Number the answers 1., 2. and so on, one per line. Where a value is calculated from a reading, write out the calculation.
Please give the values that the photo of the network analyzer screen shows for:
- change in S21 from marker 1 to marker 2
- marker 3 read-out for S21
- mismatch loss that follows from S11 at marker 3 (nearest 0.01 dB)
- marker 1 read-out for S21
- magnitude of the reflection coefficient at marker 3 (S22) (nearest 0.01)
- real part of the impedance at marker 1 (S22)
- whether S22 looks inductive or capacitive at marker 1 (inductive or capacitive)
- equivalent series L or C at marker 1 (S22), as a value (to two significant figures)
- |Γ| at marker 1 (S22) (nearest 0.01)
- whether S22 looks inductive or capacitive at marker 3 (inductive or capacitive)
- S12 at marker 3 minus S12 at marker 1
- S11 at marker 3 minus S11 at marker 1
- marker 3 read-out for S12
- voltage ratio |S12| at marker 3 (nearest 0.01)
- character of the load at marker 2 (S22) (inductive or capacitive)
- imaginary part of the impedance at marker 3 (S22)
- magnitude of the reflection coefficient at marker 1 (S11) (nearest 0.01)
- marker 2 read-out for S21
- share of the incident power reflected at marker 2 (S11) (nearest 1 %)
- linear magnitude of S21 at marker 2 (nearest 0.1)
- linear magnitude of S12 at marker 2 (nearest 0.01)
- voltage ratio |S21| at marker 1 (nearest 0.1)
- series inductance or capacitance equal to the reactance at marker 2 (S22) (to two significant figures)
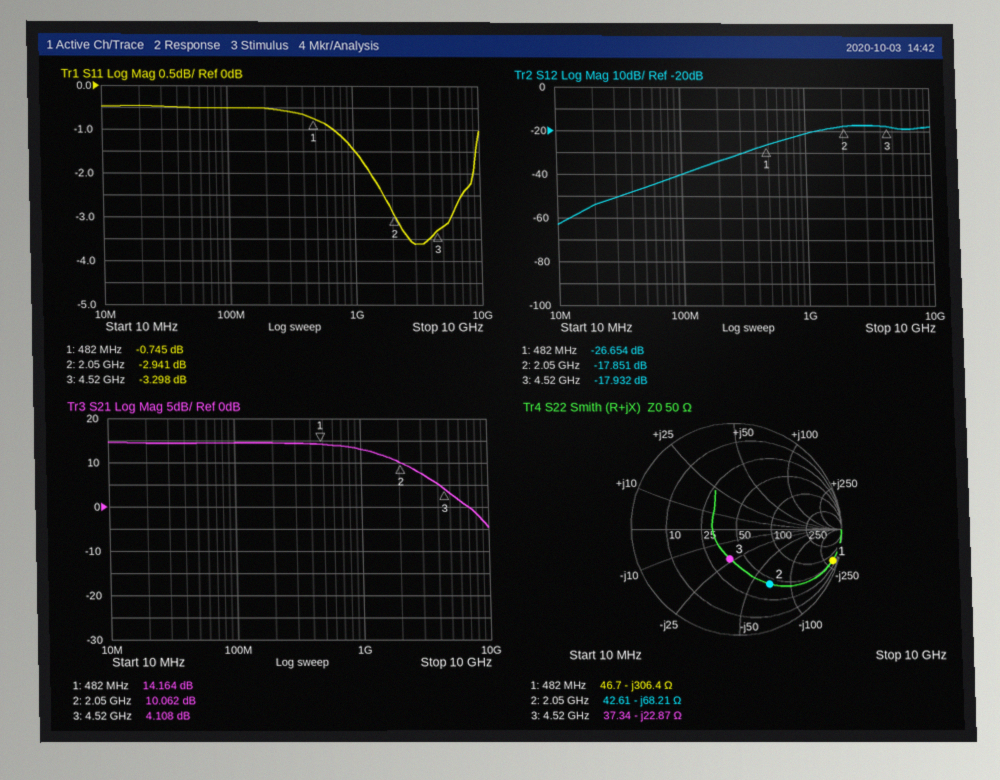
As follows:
1. 10.062 − (14.164) = -4.102 dB
2. 4.108 dB
3. −10 log10(1 − 10^(-3.298/10)) ≈ 2.74 dB
4. 14.164 dB
5. 0.29
6. 46.7 Ω
7. capacitive
8. C = 1/(2π × 482 MHz × 306.4 Ω) ≈ 1.1 pF
9. 0.95
10. capacitive
11. -17.932 − (-26.654) = 8.722 dB
12. -3.298 − (-0.745) = -2.553 dB
13. -17.932 dB
14. 10^(-17.932/20) ≈ 0.13
15. capacitive
16. -22.87 Ω
17. 10^(-0.745/20) ≈ 0.92
18. 10.062 dB
19. 10^(-2.941/10) ≈ 51 %
20. 10^(10.062/20) ≈ 3.2
21. 10^(-17.851/20) ≈ 0.13
22. 10^(14.164/20) ≈ 5.1
23. C = 1/(2π × 2.05 GHz × 68.21 Ω) ≈ 1.1 pF
